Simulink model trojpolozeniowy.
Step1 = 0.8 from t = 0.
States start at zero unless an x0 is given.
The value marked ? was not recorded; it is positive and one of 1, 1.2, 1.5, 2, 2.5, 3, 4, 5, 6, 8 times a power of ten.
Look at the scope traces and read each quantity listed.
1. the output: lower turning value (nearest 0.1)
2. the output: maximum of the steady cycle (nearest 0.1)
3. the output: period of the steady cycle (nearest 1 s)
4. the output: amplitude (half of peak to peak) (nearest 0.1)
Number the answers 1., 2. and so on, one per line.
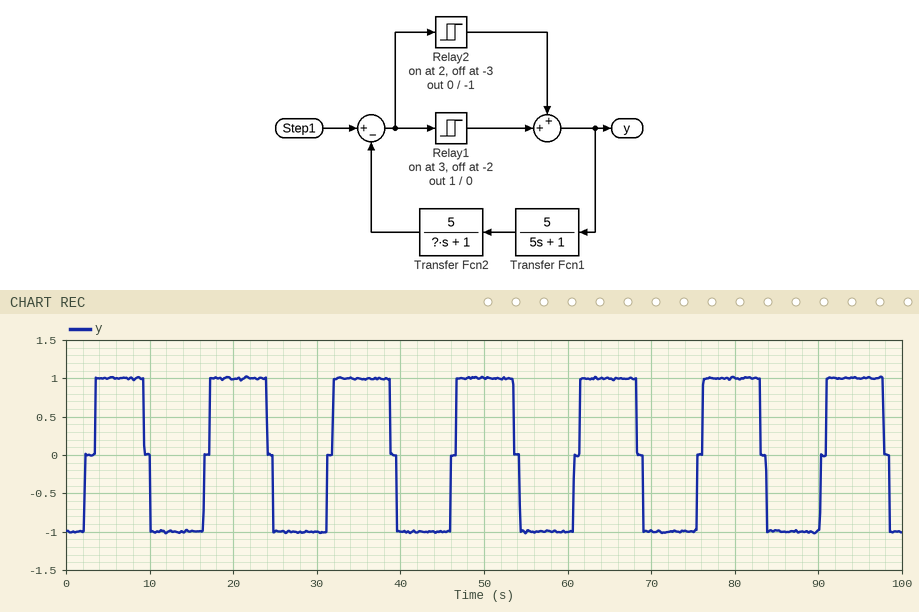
1. -1.0
2. 1.0
3. 15 s
4. 1.0
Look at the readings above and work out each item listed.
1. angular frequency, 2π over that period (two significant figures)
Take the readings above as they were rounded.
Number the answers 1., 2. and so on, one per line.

1. 0.42 rad/s
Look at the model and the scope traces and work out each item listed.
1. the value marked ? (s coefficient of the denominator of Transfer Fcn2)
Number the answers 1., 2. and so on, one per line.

1. 8
